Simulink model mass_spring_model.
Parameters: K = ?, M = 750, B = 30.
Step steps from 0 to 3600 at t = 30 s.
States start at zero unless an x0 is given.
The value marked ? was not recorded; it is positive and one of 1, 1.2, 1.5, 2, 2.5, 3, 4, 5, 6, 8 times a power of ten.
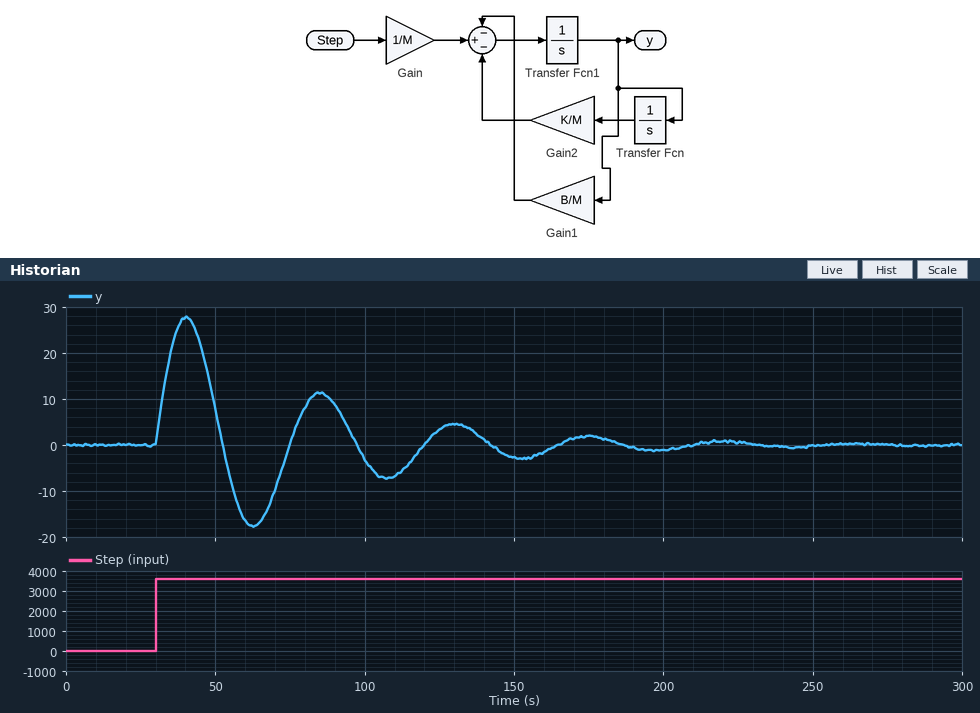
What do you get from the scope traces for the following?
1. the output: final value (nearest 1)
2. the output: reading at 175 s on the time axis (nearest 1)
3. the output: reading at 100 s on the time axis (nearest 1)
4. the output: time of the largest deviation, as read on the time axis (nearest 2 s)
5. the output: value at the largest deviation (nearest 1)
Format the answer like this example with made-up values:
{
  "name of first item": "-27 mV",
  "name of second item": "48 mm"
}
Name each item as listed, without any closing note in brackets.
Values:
{
  "the output: final value": "0",
  "the output: reading at 175 s on the time axis": "2",
  "the output: reading at 100 s on the time axis": "-3",
  "the output: time of the largest deviation, as read on the time axis": "40 s",
  "the output: value at the largest deviation": "28"
}
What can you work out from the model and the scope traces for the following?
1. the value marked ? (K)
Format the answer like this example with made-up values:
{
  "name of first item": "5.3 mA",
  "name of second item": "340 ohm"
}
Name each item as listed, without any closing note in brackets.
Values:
{
  "the value marked ?": "15"
}
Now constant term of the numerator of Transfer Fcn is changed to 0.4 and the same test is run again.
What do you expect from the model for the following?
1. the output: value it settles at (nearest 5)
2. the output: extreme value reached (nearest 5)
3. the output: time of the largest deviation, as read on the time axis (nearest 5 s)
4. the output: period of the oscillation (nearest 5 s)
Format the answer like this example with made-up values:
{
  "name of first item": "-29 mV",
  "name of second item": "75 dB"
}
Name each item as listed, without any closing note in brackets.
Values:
{
  "the output: value it settles at": "0",
  "the output: extreme value reached": "40",
  "the output: time of the largest deviation, as read on the time axis": "45 s",
  "the output: period of the oscillation": "70 s"
}
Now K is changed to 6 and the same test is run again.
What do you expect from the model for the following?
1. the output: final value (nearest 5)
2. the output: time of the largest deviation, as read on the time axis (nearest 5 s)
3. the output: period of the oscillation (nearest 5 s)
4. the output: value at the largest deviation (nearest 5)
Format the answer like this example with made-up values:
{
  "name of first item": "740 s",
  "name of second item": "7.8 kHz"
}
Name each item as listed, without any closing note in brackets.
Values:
{
  "the output: final value": "0",
  "the output: time of the largest deviation, as read on the time axis": "45 s",
  "the output: period of the oscillation": "70 s",
  "the output: value at the largest deviation": "40"
}
